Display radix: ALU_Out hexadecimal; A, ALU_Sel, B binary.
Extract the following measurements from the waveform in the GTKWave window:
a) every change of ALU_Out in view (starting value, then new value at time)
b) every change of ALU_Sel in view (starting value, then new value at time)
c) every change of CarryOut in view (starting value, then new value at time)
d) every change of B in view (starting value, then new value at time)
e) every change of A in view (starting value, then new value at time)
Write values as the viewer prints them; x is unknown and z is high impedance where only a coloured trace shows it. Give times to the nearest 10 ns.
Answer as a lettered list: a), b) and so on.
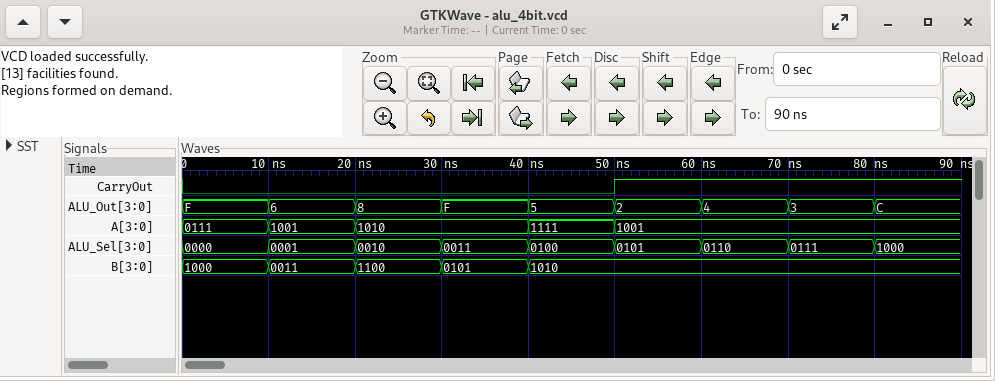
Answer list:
a) F, 6 at 10 ns, 8 at 20 ns, F at 30 ns, 5 at 40 ns, 2 at 50 ns, 4 at 60 ns, 3 at 70 ns, C at 80 ns
b) 0000, 0001 at 10 ns, 0010 at 20 ns, 0011 at 30 ns, 0100 at 40 ns, 0101 at 50 ns, 0110 at 60 ns, 0111 at 70 ns, 1000 at 80 ns
c) 0, 1 at 50 ns
d) 1000, 0011 at 10 ns, 1100 at 20 ns, 0101 at 30 ns, 1010 at 40 ns
e) 0111, 1001 at 10 ns, 1010 at 20 ns, 1111 at 40 ns, 1001 at 50 ns
